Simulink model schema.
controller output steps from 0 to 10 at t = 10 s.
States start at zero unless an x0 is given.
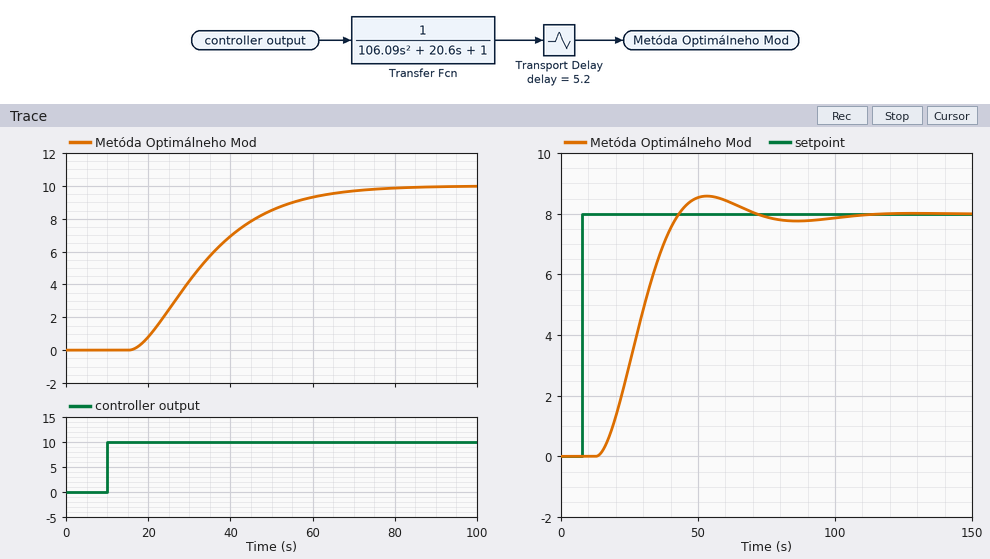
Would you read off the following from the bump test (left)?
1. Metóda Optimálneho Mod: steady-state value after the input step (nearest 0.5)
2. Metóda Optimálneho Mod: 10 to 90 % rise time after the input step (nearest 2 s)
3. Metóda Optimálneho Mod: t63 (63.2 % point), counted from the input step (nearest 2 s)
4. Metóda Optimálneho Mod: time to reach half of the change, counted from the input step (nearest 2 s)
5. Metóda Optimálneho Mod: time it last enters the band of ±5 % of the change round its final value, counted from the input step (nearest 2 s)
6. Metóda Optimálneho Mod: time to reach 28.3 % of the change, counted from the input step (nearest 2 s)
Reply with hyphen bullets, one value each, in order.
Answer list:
- 10.0
- 34 s
- 28 s
- 22 s
- 54 s
- 16 s
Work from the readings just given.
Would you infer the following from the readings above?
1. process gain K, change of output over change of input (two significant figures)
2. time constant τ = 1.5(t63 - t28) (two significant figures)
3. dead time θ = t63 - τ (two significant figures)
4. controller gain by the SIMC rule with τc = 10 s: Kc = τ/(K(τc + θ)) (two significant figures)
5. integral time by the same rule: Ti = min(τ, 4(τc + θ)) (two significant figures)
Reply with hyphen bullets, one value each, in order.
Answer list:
- 1.0
- 18 s
- 10 s
- 0.90
- 18 s
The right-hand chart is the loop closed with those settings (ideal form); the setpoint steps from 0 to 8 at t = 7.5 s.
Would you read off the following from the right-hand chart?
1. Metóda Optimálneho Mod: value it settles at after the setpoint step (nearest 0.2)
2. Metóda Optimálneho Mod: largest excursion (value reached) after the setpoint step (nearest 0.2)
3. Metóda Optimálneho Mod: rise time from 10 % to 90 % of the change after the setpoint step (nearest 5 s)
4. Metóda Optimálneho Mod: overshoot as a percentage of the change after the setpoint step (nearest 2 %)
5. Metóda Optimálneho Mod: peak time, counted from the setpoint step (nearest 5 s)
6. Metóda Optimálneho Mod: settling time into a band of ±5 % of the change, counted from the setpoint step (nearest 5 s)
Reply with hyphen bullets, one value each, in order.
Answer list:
- 8.0
- 8.6
- 20 s
- 8 %
- 45 s
- 55 s
